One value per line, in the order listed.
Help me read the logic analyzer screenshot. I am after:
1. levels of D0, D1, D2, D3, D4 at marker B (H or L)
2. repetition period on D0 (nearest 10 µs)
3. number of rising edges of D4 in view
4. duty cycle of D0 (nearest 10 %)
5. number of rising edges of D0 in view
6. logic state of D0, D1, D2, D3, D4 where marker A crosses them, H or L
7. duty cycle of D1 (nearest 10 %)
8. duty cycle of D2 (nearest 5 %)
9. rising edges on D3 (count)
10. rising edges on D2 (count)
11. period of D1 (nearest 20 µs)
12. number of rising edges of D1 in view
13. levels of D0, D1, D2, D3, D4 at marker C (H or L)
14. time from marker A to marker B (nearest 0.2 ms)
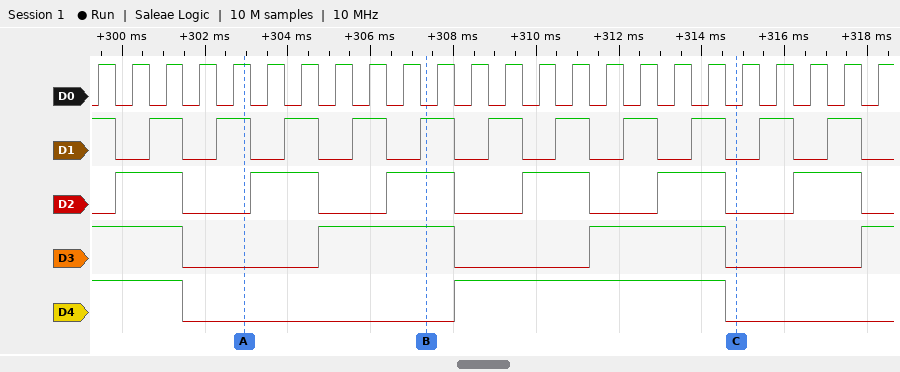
D0=L, D1=H, D2=H, D3=H, D4=L
820 µs
1
50 %
24
D0=H, D1=H, D2=L, D3=L, D4=L
50 %
50 %
3
6
1640 µs
11
D0=L, D1=L, D2=L, D3=L, D4=L
4.4 ms
